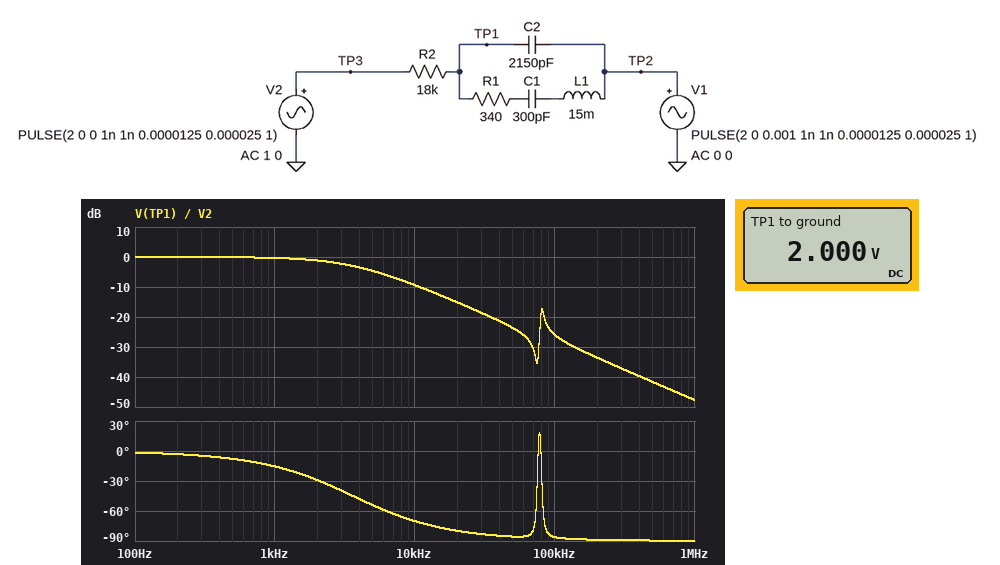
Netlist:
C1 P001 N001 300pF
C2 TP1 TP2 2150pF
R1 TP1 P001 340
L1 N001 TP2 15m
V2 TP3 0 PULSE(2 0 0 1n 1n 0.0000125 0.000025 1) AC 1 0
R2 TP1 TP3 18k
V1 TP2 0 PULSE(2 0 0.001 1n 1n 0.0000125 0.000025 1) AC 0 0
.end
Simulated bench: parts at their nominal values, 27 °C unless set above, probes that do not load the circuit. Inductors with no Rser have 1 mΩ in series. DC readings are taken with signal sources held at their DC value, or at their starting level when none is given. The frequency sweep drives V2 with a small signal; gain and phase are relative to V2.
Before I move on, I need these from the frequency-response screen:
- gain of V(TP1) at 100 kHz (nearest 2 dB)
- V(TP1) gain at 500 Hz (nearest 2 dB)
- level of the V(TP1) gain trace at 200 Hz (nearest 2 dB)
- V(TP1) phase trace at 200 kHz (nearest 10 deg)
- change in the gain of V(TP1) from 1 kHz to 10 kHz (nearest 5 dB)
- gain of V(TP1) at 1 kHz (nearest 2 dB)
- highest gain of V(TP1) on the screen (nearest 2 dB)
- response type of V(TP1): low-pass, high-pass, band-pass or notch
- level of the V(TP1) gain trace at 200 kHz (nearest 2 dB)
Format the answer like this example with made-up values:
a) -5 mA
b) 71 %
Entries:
a) -26 dB
b) 0 dB
c) 0 dB
d) -90 deg
e) -10 dB
f) 0 dB
g) 0 dB
h) low-pass
i) -34 dB
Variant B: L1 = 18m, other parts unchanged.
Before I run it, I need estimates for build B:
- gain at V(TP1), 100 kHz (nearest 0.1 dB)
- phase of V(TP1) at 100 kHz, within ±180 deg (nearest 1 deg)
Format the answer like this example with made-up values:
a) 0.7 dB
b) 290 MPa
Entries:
a) -26.6 dB
b) -87 deg
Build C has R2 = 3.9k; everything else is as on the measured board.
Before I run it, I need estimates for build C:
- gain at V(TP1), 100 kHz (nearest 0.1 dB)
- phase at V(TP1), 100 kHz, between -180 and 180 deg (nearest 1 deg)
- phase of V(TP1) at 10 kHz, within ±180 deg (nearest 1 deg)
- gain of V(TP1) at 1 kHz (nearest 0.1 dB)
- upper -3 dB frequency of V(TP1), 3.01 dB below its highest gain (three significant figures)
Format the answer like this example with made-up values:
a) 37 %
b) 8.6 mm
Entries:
a) -13.0 dB
b) -76 deg
c) -31 deg
d) 0 dB
e) 16.5 kHz
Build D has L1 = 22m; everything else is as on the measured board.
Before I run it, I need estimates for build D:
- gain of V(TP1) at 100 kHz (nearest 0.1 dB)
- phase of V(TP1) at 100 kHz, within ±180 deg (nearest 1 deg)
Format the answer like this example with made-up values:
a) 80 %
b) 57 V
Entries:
a) -26.9 dB
b) -87 deg
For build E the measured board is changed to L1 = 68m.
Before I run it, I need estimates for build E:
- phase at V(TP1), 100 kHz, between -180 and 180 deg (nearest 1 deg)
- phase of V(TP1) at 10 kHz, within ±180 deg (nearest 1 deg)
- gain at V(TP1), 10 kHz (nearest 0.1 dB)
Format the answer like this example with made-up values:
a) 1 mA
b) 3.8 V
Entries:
a) -88 deg
b) -70 deg
c) -9.5 dB
